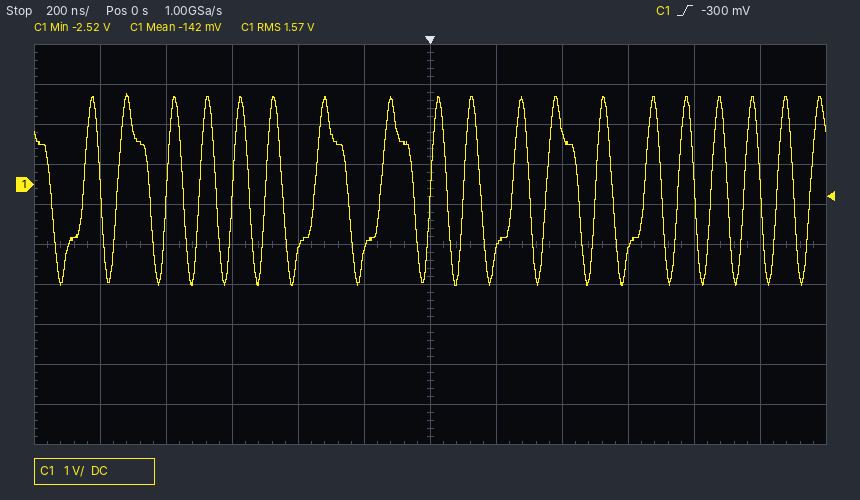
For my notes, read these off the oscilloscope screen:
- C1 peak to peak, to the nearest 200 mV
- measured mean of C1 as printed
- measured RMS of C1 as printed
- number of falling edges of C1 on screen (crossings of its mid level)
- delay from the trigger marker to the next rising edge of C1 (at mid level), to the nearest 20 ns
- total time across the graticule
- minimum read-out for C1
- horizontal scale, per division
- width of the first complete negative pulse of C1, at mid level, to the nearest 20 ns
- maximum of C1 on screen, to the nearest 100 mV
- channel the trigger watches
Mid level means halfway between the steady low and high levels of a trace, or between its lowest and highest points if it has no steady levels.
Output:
4.8 V
-142 mV
1.57 V
19
100 ns
2.4 µs
-2.52 V
200 ns
100 ns
2.3 V
C1
